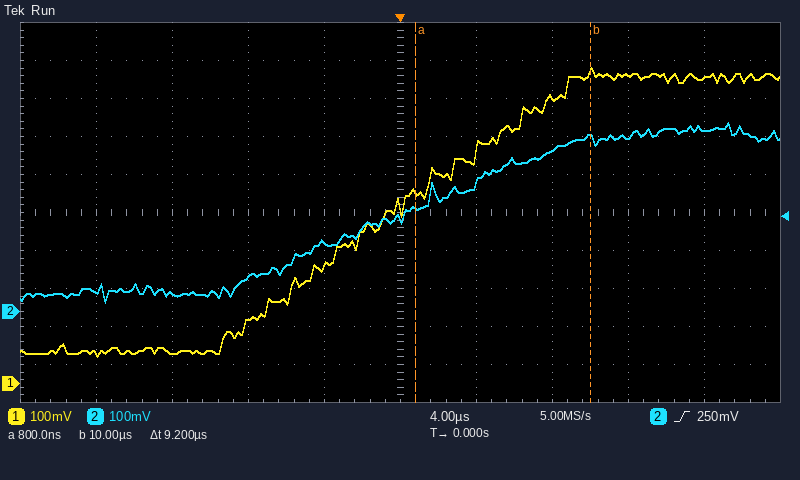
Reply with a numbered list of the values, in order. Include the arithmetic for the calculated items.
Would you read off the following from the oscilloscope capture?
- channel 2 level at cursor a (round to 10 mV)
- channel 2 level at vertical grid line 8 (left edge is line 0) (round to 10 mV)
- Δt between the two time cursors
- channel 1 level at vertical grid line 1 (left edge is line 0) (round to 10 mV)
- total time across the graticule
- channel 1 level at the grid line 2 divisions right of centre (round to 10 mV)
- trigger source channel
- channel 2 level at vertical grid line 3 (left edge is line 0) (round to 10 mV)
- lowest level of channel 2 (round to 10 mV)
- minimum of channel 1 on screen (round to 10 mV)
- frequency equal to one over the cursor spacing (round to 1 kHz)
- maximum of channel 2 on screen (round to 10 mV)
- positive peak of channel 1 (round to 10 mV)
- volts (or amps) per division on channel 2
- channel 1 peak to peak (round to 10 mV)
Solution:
1. 270 mV
2. 460 mV
3. 9.2 µs
4. 80 mV
5. 40 µs
6. 750 mV
7. channel 2
8. 90 mV
9. 20 mV
10. 70 mV
11. 1 / 9.2 µs ≈ 109 kHz
12. 500 mV
13. 830 mV
14. 100 mV
15. 830 mV − (70 mV) = 760 mV
